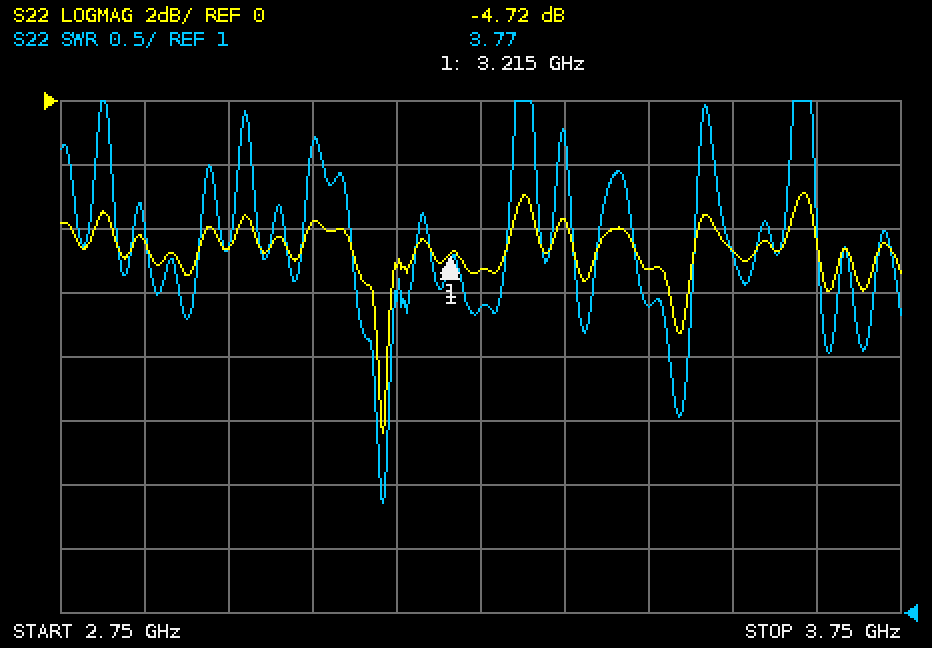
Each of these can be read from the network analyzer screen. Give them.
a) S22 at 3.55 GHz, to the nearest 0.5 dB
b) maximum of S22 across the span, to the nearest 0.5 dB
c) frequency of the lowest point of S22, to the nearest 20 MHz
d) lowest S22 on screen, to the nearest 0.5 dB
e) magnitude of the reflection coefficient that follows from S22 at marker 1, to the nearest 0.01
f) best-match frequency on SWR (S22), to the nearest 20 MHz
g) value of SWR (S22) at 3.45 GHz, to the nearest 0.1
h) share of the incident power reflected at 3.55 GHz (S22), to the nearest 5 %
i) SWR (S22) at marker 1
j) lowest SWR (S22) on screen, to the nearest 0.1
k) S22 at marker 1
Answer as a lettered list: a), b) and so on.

a) -4.5 dB
b) -3.0 dB
c) 3.14 GHz
d) -10.5 dB
e) 0.58
f) 3.14 GHz
g) 3.4
h) 35 %
i) 3.77
j) 1.9
k) -4.72 dB
